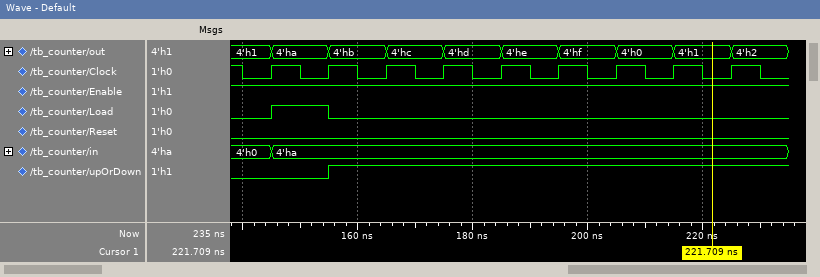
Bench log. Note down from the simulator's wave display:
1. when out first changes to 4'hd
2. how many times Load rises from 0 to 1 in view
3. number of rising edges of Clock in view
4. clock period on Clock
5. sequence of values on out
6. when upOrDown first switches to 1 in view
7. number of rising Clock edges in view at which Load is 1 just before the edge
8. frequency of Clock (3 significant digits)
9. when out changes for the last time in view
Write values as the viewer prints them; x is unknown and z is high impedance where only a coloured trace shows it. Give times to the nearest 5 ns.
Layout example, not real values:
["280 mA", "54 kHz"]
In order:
["175 ns", "1", "9", "10 ns", "4'h1, 4'ha, 4'hb, 4'hc, 4'hd, 4'he, 4'hf, 4'h0, 4'h1, 4'h2", "155 ns", "1", "100 MHz", "225 ns"]
